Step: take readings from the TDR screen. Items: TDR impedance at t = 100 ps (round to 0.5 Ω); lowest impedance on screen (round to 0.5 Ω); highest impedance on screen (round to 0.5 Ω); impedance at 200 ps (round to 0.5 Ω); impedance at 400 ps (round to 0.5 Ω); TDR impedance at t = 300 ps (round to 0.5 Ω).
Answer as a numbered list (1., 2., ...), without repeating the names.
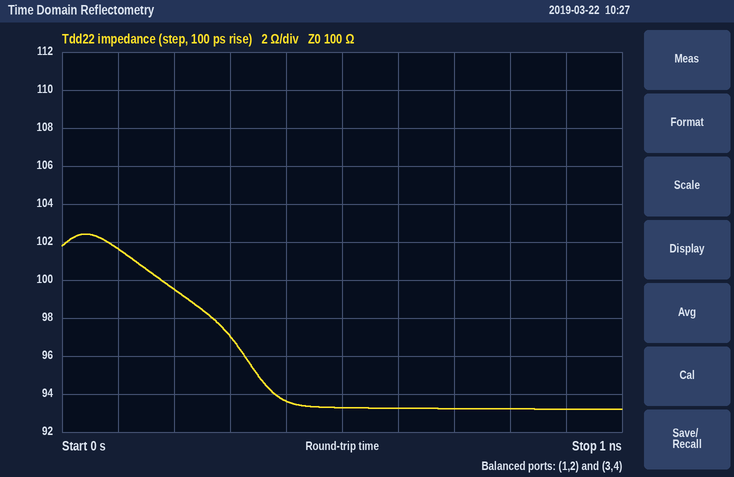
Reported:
1. 101.5 Ω
2. 93.0 Ω
3. 102.5 Ω
4. 99.5 Ω
5. 93.5 Ω
6. 97.0 Ω
